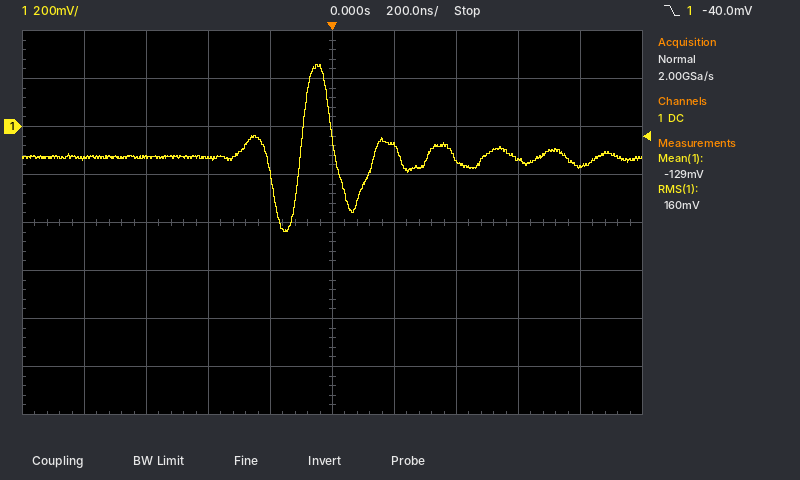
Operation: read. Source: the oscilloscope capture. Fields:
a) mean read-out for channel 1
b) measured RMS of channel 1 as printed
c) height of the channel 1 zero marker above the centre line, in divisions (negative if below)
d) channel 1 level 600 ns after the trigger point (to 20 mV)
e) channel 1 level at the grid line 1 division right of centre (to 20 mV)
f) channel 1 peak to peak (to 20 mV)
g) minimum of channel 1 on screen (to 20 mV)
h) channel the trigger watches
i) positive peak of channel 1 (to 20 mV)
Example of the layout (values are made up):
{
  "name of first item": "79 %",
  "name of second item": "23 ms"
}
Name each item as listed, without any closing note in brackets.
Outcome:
{
  "mean read-out for channel 1": "-129 mV",
  "measured RMS of channel 1 as printed": "160 mV",
  "height of the channel 1 zero marker above the centre line, in divisions": "+2.0 div",
  "channel 1 level 600 ns after the trigger point": "-140 mV",
  "channel 1 level at the grid line 1 division right of centre": "-80 mV",
  "channel 1 peak to peak": "700 mV",
  "minimum of channel 1 on screen": "-440 mV",
  "channel the trigger watches": "channel 1",
  "positive peak of channel 1": "260 mV"
}
